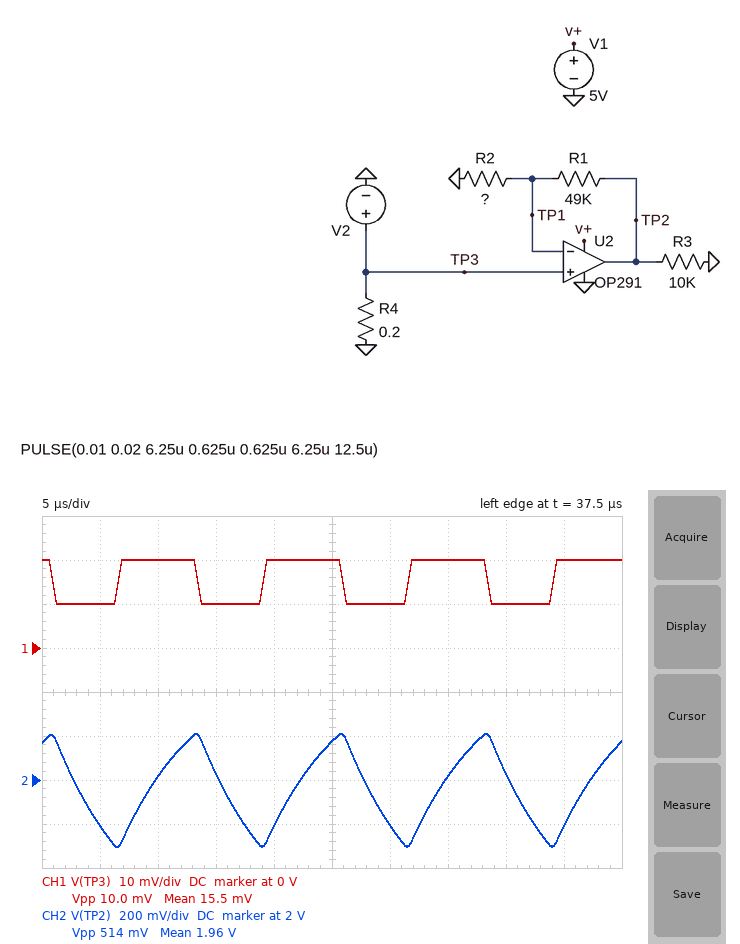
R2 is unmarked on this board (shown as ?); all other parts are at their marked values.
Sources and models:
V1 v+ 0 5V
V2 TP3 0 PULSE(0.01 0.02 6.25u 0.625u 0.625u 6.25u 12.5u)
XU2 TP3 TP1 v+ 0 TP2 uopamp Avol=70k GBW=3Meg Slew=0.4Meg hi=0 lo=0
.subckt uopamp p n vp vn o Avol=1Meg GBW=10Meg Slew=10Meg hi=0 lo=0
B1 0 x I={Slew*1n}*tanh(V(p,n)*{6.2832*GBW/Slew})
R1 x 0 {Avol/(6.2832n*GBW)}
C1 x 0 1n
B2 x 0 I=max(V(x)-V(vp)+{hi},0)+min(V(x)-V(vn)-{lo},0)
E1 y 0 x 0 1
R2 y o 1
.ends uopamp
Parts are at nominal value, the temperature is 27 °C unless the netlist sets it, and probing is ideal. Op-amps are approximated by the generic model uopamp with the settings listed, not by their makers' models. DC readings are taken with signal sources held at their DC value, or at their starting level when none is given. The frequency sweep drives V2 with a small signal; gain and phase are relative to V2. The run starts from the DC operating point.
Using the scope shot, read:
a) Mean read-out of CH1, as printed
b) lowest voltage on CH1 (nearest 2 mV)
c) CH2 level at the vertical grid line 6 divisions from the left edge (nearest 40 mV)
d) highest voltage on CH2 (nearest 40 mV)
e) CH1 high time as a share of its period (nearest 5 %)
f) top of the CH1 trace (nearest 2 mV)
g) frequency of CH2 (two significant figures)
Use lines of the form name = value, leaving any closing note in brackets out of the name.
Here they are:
Mean read-out of CH1, as printed = 15.5 mV
lowest voltage on CH1 = 10 mV
CH2 level at the vertical grid line 6 divisions from the left edge = 1.80 V
highest voltage on CH2 = 2.20 V
CH1 high time as a share of its period = 55 %
top of the CH1 trace = 20 mV
frequency of CH2 = 80 kHz
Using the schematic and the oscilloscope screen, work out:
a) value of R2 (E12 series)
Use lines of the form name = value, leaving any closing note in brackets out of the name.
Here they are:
value of R2 = 390 Ω
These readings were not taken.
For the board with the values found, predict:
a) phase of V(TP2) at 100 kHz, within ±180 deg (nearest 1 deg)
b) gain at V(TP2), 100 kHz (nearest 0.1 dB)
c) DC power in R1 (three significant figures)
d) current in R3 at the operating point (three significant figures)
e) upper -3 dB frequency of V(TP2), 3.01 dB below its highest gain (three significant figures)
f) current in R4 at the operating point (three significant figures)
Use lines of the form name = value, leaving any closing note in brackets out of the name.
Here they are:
phase of V(TP2) at 100 kHz, within ±180 deg = -77 deg
gain at V(TP2), 100 kHz = 29.3 dB
DC power in R1 = 32.1 µW
current in R3 at the operating point = 126 µA
upper -3 dB frequency of V(TP2), 3.01 dB below its highest gain = 23.7 kHz
current in R4 at the operating point = 50.0 mA
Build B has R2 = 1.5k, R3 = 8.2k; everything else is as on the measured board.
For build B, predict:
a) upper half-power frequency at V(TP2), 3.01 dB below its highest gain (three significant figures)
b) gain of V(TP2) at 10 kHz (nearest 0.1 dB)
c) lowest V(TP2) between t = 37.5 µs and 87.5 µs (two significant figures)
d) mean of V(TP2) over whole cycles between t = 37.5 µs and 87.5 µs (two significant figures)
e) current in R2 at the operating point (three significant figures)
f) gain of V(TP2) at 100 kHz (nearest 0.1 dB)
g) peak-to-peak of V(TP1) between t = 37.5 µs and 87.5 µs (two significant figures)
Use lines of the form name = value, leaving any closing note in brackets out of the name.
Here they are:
upper half-power frequency at V(TP2), 3.01 dB below its highest gain = 89.1 kHz
gain of V(TP2) at 10 kHz = 30.5 dB
lowest V(TP2) between t = 37.5 µs and 87.5 µs = 350 mV
mean of V(TP2) over whole cycles between t = 37.5 µs and 87.5 µs = 520 mV
current in R2 at the operating point = 6.66 µA
gain of V(TP2) at 100 kHz = 27.0 dB
peak-to-peak of V(TP1) between t = 37.5 µs and 87.5 µs = 9.2 mV
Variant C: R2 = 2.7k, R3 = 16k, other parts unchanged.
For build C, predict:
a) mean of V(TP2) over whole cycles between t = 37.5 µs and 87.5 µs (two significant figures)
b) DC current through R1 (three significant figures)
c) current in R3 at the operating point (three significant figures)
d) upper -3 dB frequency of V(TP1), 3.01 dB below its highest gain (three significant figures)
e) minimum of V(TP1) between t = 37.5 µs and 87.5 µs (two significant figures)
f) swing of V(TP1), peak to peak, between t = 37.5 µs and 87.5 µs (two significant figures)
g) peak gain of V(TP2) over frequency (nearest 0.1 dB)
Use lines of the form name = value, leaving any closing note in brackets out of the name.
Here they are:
mean of V(TP2) over whole cycles between t = 37.5 µs and 87.5 µs = 300 mV
DC current through R1 = 3.70 µA
current in R3 at the operating point = 12.0 µA
upper -3 dB frequency of V(TP1), 3.01 dB below its highest gain = 157 kHz
minimum of V(TP1) between t = 37.5 µs and 87.5 µs = 10 mV
swing of V(TP1), peak to peak, between t = 37.5 µs and 87.5 µs = 9.9 mV
peak gain of V(TP2) over frequency = 25.6 dB
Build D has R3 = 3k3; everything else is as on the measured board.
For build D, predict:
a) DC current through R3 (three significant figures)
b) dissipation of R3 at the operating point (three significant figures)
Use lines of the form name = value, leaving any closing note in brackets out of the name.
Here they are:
DC current through R3 = 383 µA
dissipation of R3 at the operating point = 484 µW
